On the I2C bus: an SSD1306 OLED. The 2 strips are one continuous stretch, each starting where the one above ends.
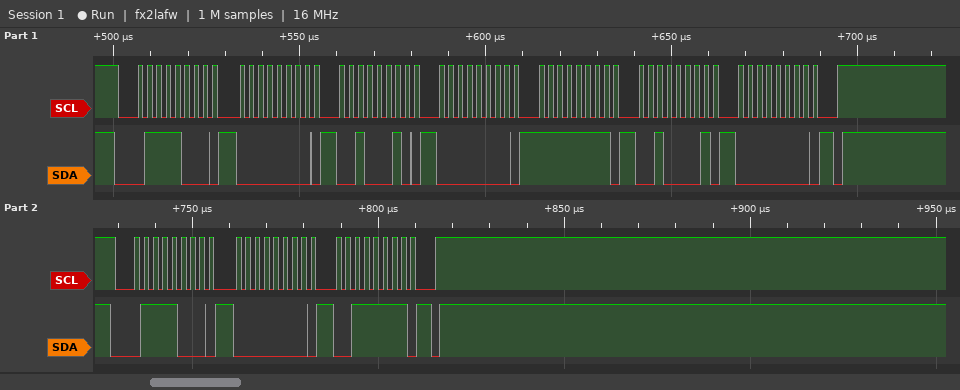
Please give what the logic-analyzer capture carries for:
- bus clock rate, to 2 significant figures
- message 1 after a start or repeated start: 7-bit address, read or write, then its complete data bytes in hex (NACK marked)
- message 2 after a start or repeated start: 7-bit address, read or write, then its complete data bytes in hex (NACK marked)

400 kHz
0x3C write: 00 22 00 FF 21 00
0x3C write: 00 3F
